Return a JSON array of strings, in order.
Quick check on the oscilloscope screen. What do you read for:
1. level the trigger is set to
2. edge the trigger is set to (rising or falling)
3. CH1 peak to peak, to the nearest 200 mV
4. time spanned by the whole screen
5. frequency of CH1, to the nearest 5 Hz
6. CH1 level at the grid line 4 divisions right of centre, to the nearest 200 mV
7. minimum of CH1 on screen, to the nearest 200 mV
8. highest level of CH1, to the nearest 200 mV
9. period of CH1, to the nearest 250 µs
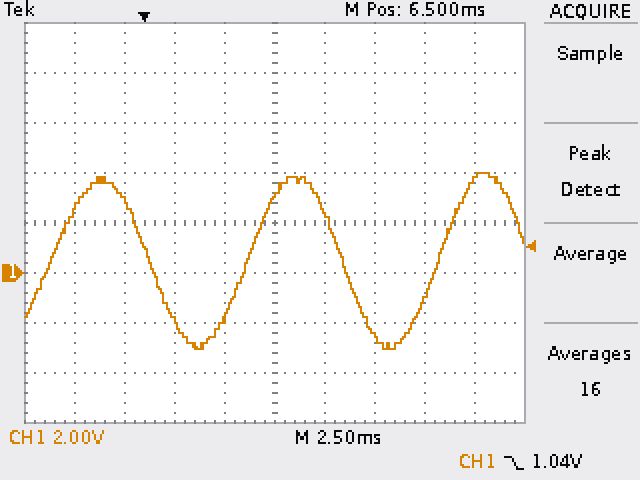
["1.04 V", "falling", "7.0 V", "25 ms", "105 Hz", "3.8 V", "-3.0 V", "4.0 V", "9.75 ms"]
